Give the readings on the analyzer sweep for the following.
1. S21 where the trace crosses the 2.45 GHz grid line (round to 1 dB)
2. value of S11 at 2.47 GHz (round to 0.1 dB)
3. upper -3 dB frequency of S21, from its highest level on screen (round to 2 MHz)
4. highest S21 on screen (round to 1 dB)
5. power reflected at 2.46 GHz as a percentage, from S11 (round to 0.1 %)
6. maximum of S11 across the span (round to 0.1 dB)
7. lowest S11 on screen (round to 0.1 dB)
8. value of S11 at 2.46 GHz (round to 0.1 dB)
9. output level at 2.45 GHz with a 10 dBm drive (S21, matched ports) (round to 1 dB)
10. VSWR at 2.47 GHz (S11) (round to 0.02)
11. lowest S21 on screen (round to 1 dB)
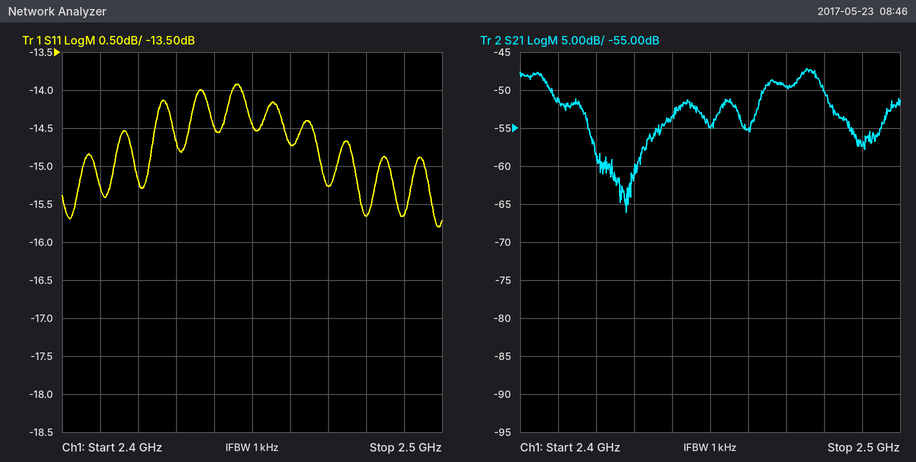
-55 dB
-15.3 dB
2.480 GHz
-47 dB
3.4 %
-13.9 dB
-15.8 dB
-14.7 dB
-45 dBm
1.42
-66 dB
